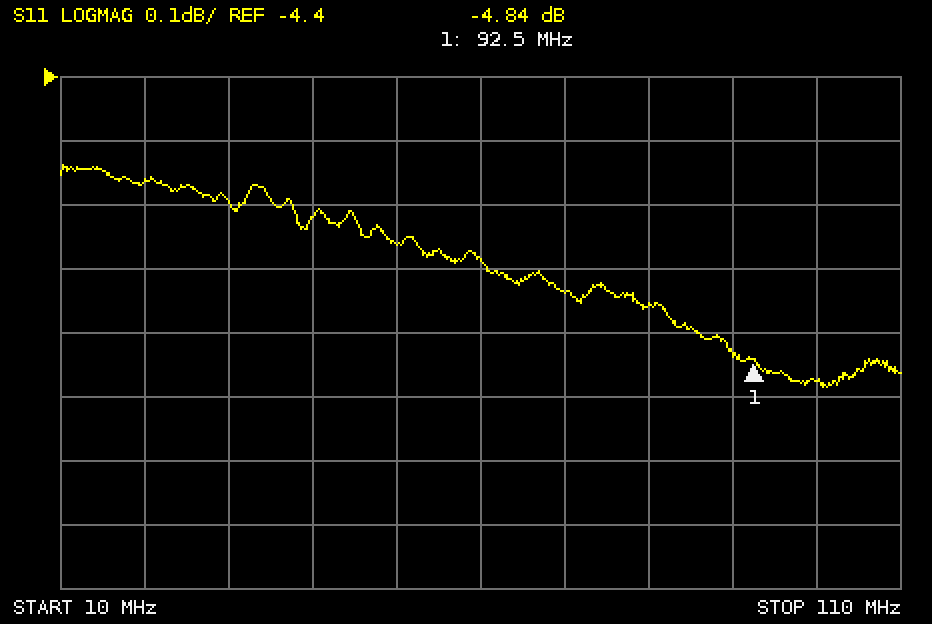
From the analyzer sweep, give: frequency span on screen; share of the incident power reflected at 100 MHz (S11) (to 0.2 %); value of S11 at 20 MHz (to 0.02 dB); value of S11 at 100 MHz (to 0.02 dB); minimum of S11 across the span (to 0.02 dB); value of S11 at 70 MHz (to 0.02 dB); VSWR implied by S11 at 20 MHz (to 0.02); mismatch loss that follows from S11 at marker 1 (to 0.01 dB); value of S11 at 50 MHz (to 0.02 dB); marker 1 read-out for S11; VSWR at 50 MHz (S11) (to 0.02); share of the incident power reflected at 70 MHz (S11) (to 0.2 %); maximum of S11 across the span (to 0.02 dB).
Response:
100 MHz
32.6 %
-4.56 dB
-4.88 dB
-4.88 dB
-4.74 dB
3.90
1.73 dB
-4.66 dB
-4.84 dB
3.82
33.6 %
-4.54 dB
